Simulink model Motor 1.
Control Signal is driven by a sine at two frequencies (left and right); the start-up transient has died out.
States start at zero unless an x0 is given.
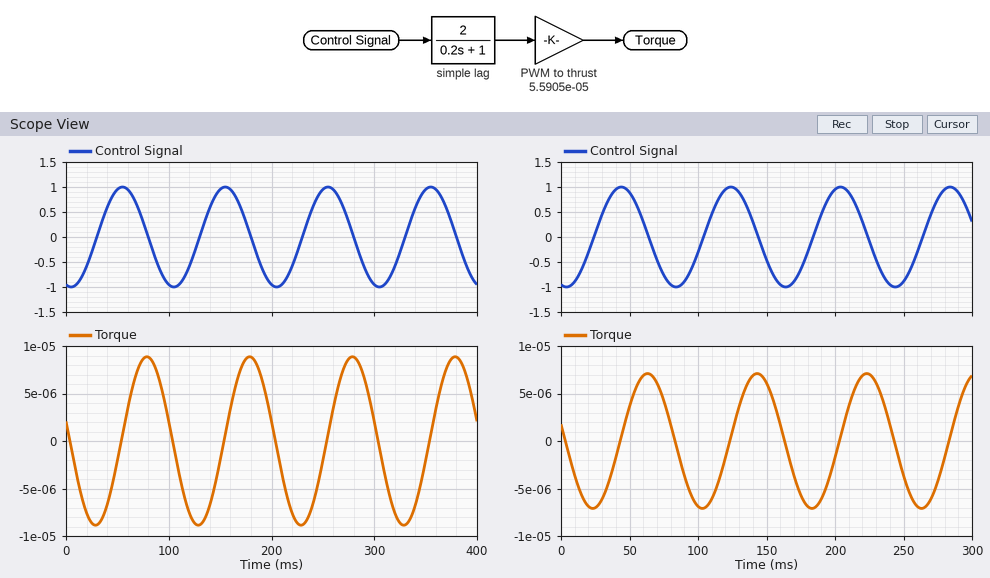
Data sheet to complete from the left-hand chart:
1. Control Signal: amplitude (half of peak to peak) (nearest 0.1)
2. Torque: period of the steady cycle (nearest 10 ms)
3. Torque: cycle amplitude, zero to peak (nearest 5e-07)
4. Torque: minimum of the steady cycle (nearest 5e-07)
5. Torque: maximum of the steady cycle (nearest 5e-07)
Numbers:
1.0
100 ms
0.0000090
-0.0000090
0.0000090
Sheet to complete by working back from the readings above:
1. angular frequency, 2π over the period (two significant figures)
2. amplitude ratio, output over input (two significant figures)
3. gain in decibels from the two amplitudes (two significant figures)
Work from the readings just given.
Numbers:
0.063 rad/ms
0.0000090
-100 dB
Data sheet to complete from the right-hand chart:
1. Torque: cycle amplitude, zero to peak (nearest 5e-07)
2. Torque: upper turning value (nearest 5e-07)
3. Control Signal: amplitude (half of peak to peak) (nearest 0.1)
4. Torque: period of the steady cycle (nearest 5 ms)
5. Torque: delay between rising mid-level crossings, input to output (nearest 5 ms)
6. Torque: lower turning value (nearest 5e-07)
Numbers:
0.0000070
0.0000070
1.0
80 ms
20 ms
-0.0000070
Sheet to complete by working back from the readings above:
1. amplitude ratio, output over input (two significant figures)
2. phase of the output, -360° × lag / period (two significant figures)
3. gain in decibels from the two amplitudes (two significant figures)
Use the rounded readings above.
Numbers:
0.0000070
-90°
-100 dB
